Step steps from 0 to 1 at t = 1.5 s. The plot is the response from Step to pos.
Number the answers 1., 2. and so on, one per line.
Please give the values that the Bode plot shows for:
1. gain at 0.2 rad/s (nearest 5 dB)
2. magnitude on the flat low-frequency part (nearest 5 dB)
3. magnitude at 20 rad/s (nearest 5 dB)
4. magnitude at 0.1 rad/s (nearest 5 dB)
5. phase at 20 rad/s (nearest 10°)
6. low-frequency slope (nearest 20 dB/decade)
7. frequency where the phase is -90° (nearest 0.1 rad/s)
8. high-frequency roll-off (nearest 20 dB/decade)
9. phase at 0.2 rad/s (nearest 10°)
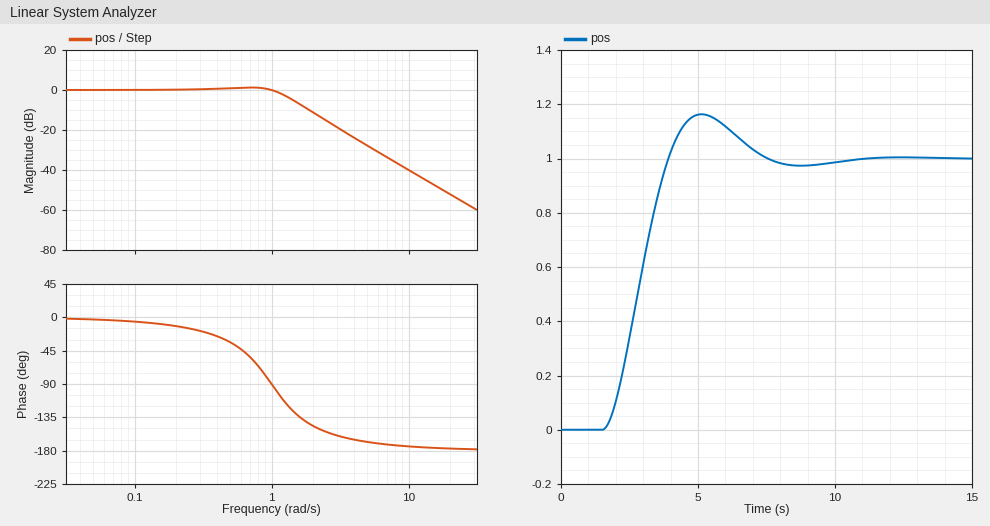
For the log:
1. 0 dB
2. 0 dB
3. -50 dB
4. 0 dB
5. -180°
6. 0 dB/decade
7. 1.0 rad/s
8. -40 dB/decade
9. -10°
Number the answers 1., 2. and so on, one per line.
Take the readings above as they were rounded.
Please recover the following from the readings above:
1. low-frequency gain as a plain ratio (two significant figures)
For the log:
1. 1.0
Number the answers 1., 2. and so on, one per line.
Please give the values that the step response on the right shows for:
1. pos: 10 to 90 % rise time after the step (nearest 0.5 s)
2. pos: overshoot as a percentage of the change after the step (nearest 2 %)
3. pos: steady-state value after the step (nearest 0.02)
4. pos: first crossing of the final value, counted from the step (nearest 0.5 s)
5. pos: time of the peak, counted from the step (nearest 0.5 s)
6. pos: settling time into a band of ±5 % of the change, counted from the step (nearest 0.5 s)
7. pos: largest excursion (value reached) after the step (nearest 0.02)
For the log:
1. 1.5 s
2. 16 %
3. 1.00
4. 2.5 s
5. 3.5 s
6. 5.5 s
7. 1.16
